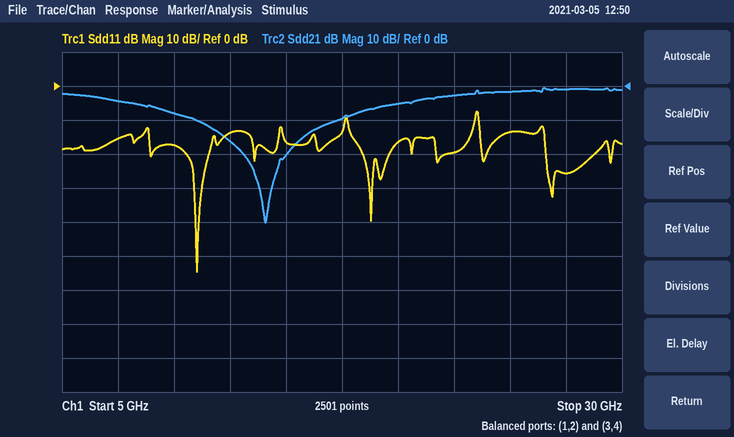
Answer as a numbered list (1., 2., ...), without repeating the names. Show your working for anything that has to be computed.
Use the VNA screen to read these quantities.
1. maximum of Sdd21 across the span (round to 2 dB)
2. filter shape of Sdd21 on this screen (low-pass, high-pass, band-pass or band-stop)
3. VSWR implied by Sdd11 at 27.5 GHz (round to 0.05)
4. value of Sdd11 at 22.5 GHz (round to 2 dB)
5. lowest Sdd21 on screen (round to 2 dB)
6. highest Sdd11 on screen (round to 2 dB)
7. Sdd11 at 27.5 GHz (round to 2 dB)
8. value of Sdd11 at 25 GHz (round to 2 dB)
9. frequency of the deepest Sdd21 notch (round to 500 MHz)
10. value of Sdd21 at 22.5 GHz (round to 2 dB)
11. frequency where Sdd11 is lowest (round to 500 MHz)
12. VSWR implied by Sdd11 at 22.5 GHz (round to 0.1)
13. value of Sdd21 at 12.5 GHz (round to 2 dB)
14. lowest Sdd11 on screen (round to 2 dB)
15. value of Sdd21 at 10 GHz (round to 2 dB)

1. 0 dB
2. band-stop
3. |Γ| = 10^(-26/20) = 0.0501; VSWR = (1 + 0.0501)/(1 − 0.0501) ≈ 1.11, so 1.10 to the nearest 0.05
4. -20 dB
5. -40 dB
6. -8 dB
7. -26 dB
8. -14 dB
9. 14.0 GHz
10. -2 dB
11. 11.0 GHz
12. |Γ| = 10^(-20/20) = 0.1000; VSWR = (1 + 0.1000)/(1 − 0.1000) ≈ 1.2
13. -16 dB
14. -54 dB
15. -8 dB
